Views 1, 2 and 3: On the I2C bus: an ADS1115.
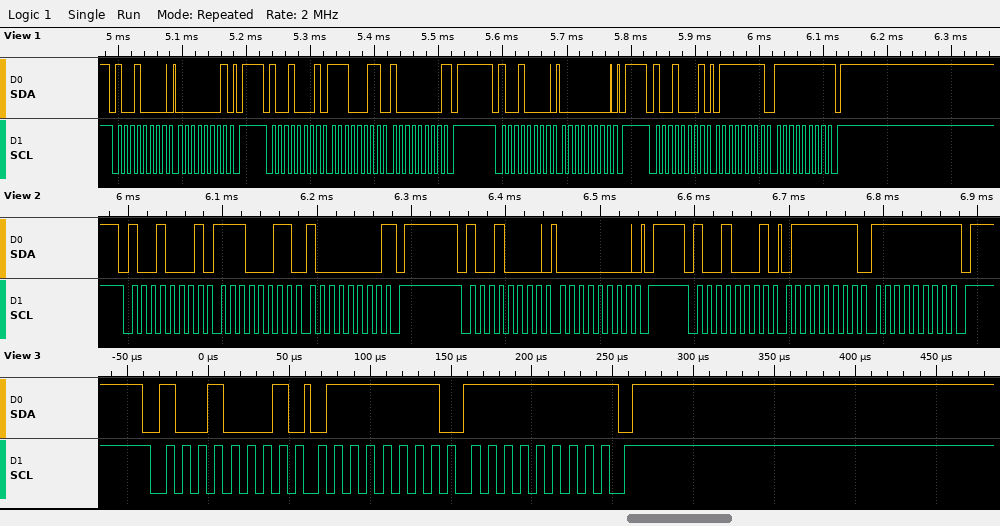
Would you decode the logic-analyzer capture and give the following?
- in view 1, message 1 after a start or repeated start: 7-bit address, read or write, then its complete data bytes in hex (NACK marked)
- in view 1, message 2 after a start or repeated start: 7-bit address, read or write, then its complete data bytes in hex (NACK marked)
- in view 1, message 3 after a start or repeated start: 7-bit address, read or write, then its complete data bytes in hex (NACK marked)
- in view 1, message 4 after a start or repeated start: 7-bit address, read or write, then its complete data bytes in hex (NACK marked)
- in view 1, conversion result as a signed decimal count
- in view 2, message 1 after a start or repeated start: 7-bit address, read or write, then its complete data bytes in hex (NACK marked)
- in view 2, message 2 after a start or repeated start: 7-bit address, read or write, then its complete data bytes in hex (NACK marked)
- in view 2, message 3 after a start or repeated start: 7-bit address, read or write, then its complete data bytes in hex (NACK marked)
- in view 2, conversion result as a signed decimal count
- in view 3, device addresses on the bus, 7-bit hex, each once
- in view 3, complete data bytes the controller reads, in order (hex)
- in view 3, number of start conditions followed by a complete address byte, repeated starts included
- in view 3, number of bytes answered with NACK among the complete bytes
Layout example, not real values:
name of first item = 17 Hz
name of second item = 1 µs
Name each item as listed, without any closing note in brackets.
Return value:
in view 1, message 1 after a start or repeated start: 7-bit address, read or write, then its complete data bytes in hex = 0x48 write: 01
in view 1, message 2 after a start or repeated start: 7-bit address, read or write, then its complete data bytes in hex = 0x48 read: E3 80 NACK
in view 1, message 3 after a start or repeated start: 7-bit address, read or write, then its complete data bytes in hex = 0x48 write: 00
in view 1, message 4 after a start or repeated start: 7-bit address, read or write, then its complete data bytes in hex = 0x48 read: 7F FF NACK
in view 1, conversion result as a signed decimal count = 32767
in view 2, message 1 after a start or repeated start: 7-bit address, read or write, then its complete data bytes in hex = 0x48 read: E3 80 NACK
in view 2, message 2 after a start or repeated start: 7-bit address, read or write, then its complete data bytes in hex = 0x48 write: 00
in view 2, message 3 after a start or repeated start: 7-bit address, read or write, then its complete data bytes in hex = 0x48 read: 7F FF NACK
in view 2, conversion result as a signed decimal count = 32767
in view 3, device addresses on the bus, 7-bit hex, each once = 0x48
in view 3, complete data bytes the controller reads, in order = 7F FF
in view 3, number of start conditions followed by a complete address byte, repeated starts included = 1
in view 3, number of bytes answered with NACK among the complete bytes = 1
